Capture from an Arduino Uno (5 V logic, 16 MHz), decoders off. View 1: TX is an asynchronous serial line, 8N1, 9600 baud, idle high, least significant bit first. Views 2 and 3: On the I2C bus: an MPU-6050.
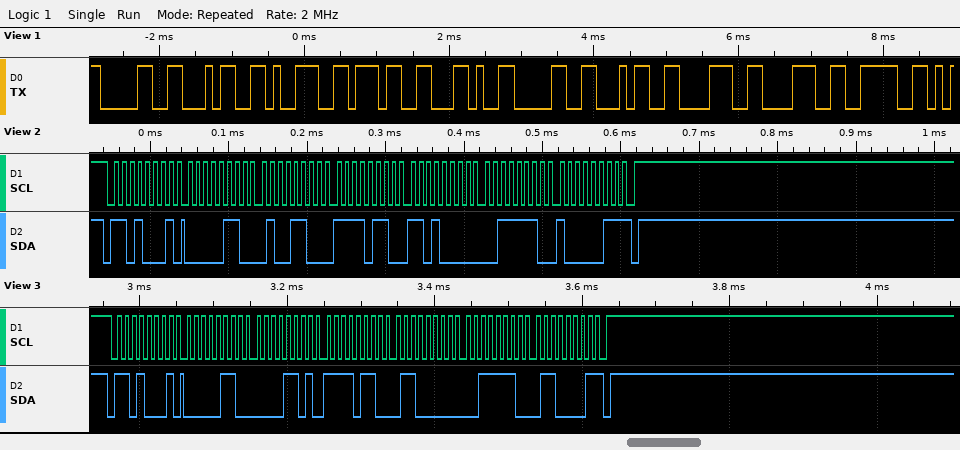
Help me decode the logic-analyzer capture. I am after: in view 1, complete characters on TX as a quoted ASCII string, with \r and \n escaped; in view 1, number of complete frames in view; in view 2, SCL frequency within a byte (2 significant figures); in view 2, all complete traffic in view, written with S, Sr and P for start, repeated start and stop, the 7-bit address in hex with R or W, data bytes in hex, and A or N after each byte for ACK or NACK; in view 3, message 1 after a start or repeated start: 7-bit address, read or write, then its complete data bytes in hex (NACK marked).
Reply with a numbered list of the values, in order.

1. "0497,0488>"
2. 10
3. 100 kHz
4. S 68R A 06 A 4C A F6 A D0 A 3E A 83 N P
5. 0x68 read: 06 0D F6 60 3E 61 NACK
